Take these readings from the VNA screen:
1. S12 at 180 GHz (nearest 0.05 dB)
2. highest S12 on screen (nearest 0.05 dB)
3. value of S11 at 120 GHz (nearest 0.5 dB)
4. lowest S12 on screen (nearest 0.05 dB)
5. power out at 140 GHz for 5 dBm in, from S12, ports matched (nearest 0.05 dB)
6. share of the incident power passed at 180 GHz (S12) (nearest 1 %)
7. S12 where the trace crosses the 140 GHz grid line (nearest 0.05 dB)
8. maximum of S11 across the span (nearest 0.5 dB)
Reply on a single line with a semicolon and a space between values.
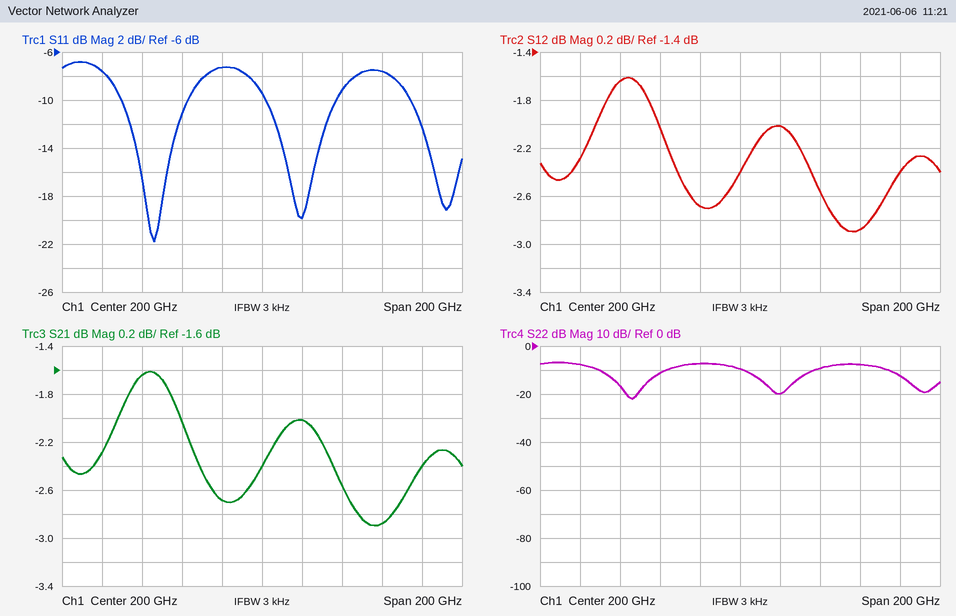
-2.70 dB; -1.60 dB; -7.5 dB; -2.90 dB; 3.35 dBm; 54 %; -1.65 dB; -7.0 dB
